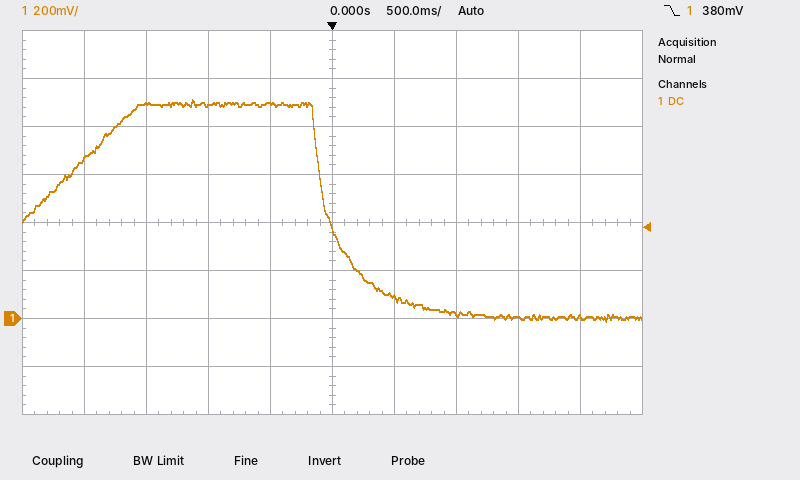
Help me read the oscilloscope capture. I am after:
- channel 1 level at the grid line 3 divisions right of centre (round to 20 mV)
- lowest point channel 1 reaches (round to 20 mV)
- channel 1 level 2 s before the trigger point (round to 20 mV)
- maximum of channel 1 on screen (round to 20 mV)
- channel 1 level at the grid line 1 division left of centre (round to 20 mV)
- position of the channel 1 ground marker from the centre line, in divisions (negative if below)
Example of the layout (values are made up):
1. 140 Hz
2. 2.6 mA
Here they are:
1. 0 mV
2. -20 mV
3. 660 mV
4. 920 mV
5. 900 mV
6. -2.0 div
